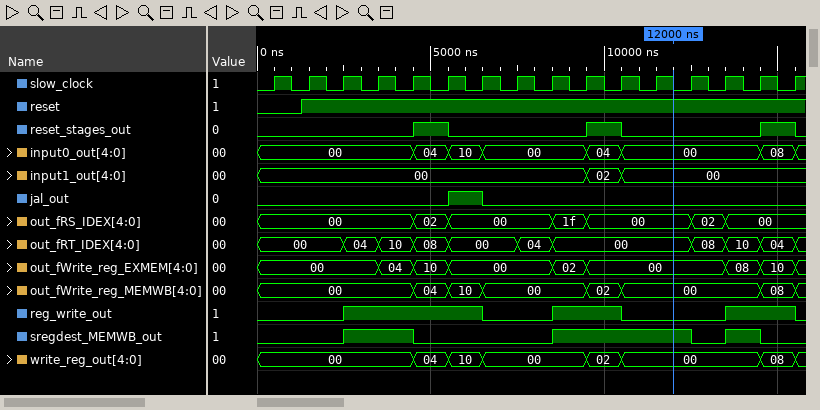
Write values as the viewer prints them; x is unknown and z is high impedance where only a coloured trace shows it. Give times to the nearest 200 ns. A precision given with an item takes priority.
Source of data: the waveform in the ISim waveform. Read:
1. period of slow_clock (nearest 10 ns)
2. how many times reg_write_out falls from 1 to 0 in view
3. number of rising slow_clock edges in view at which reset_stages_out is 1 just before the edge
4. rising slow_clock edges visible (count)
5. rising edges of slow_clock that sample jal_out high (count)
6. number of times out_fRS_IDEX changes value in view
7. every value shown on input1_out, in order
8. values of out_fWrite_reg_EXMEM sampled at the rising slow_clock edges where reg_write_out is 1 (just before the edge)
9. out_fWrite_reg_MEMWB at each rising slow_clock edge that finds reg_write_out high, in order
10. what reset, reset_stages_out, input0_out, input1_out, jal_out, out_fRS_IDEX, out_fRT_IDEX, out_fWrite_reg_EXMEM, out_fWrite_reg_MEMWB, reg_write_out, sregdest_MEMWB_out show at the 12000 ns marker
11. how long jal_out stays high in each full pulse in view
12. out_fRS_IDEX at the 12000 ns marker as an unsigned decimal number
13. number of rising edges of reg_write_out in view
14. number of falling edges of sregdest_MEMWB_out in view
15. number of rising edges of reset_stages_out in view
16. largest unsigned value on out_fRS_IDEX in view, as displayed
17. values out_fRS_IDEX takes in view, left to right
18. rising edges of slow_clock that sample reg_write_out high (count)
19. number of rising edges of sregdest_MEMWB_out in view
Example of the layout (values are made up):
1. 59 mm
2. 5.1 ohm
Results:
1. 1000 ns
2. 3
3. 3
4. 16
5. 1
6. 6
7. 00, 02, 00
8. 00, 04, 10, 00, 02, 00, 08, 10
9. 00, 00, 04, 10, 00, 02, 00, 08
10. reset=1, reset_stages_out=0, input0_out=00, input1_out=00, jal_out=0, out_fRS_IDEX=00, out_fRT_IDEX=00, out_fWrite_reg_EXMEM=00, out_fWrite_reg_MEMWB=00, reg_write_out=0, sregdest_MEMWB_out=1
11. 1000 ns
12. 0
13. 3
14. 3
15. 3
16. 1f
17. 00, 02, 00, 1f, 00, 02, 00
18. 8
19. 3
